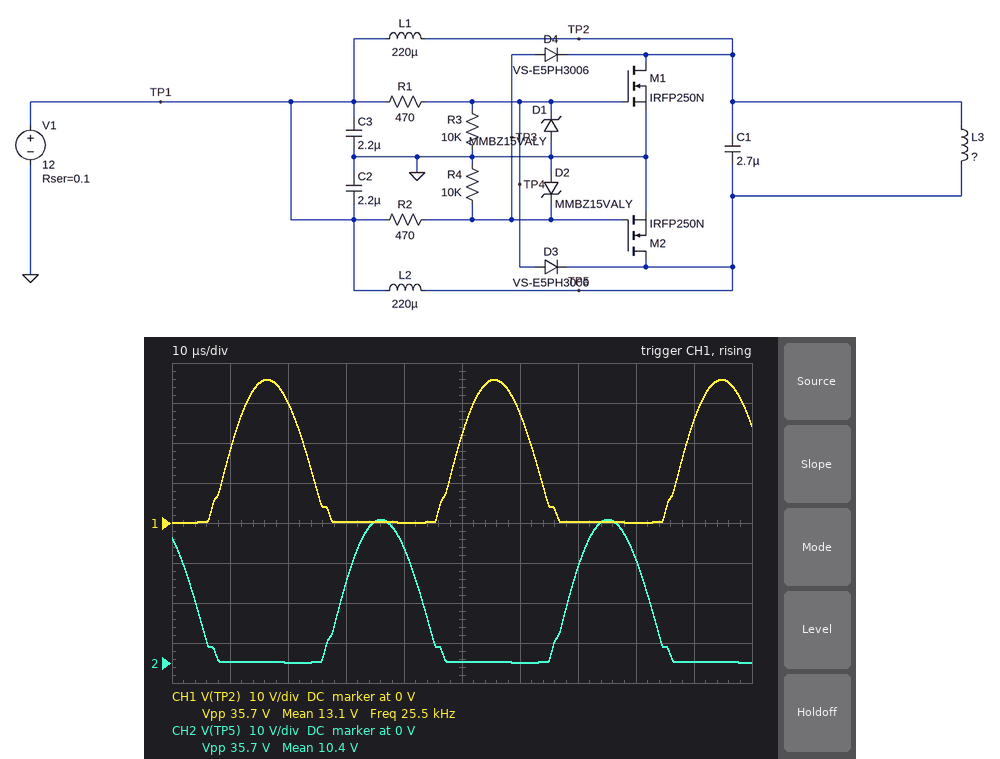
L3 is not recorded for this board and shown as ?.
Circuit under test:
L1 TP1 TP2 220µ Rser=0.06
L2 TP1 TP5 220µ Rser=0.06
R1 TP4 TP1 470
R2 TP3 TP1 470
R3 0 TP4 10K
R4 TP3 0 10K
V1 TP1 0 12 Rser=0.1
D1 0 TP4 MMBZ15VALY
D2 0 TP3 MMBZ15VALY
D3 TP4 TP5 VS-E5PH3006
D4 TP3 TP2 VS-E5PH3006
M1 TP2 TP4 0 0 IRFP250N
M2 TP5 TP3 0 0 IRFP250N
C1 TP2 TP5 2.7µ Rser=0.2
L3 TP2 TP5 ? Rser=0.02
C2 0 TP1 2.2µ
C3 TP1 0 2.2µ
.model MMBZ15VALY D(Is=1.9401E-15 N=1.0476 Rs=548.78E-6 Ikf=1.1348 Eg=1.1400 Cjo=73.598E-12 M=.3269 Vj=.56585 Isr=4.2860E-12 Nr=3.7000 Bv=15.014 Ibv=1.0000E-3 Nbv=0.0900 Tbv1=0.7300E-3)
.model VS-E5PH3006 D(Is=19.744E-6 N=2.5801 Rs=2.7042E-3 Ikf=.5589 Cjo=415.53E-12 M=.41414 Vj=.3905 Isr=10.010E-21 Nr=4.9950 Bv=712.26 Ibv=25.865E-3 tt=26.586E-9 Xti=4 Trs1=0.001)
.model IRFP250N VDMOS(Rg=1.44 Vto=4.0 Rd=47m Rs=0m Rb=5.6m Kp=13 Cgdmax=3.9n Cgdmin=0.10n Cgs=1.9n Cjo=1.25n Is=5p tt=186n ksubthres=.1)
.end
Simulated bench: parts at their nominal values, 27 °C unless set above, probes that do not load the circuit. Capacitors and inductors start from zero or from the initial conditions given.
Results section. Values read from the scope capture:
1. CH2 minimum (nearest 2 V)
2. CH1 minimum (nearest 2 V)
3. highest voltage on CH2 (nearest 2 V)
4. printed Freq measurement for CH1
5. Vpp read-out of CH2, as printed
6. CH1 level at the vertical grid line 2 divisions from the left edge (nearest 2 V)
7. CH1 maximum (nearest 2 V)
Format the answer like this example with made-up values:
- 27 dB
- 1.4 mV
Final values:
- 0 V
- 0 V
- 36 V
- 25.5 kHz
- 35.7 V
- 30 V
- 36 V
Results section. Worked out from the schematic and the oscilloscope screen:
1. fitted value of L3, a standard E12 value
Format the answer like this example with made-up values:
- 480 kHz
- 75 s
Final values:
- 15 µH
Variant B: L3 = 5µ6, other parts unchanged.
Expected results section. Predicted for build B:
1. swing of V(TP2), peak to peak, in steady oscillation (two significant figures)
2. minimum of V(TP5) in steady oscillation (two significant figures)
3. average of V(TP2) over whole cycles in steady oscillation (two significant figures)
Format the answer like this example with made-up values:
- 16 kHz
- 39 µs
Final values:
- 33 V
- 320 mV
- 11 V
